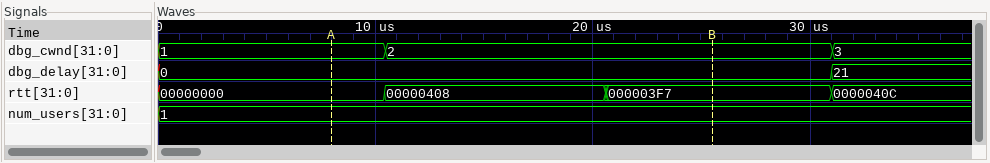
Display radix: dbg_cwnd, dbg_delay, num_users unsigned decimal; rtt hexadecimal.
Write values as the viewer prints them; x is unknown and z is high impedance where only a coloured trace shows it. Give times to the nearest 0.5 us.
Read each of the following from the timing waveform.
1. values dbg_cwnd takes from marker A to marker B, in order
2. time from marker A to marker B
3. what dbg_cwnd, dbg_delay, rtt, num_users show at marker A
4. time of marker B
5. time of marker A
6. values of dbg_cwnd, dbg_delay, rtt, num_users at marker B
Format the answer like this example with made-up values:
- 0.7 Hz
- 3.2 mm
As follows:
- 1, 2
- 17.5 us
- dbg_cwnd=1, dbg_delay=0, rtt=00000000, num_users=1
- 25.5 us
- 8 us
- dbg_cwnd=2, dbg_delay=0, rtt=000003F7, num_users=1
